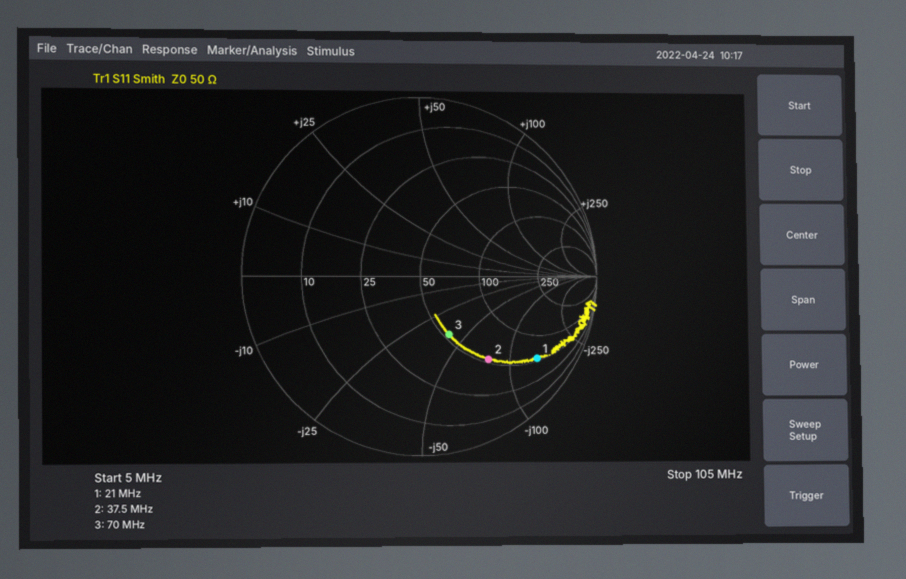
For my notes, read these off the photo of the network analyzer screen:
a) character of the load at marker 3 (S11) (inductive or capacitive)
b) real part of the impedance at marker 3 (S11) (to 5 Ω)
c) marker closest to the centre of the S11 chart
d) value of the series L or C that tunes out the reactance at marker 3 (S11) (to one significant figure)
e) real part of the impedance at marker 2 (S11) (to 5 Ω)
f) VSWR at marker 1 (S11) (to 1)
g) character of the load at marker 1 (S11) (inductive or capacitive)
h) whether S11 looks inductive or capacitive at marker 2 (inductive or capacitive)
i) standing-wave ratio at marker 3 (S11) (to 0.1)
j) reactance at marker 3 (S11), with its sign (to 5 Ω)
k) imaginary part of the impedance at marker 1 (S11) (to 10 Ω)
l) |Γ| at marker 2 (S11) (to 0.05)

capacitive
55 Ω
marker 3
90 nH
55 Ω
9
capacitive
capacitive
2.1
-40 Ω
-140 Ω
0.60
